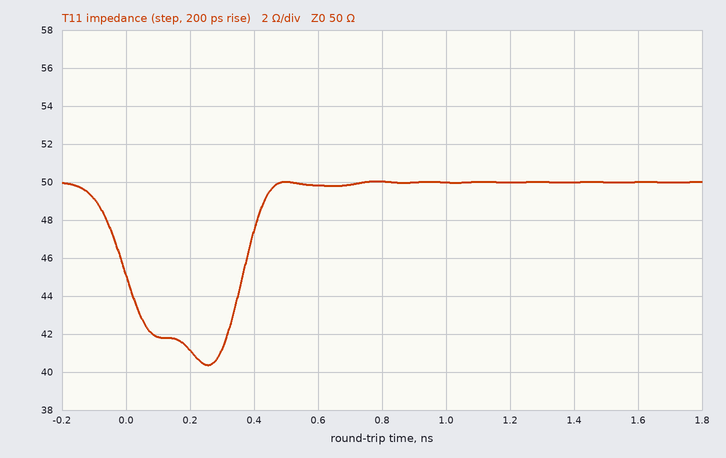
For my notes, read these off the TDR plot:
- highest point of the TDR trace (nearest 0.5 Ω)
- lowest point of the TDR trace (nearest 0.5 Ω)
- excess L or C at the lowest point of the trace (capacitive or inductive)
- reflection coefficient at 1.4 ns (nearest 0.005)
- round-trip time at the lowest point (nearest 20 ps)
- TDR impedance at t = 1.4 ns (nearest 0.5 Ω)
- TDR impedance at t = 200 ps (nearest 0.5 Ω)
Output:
50.0 Ω
40.5 Ω
capacitive
0.000
260 ps
50.0 Ω
41.0 Ω
